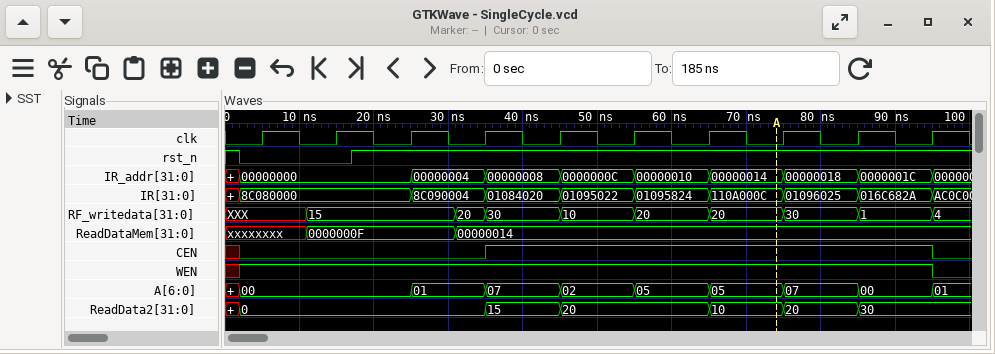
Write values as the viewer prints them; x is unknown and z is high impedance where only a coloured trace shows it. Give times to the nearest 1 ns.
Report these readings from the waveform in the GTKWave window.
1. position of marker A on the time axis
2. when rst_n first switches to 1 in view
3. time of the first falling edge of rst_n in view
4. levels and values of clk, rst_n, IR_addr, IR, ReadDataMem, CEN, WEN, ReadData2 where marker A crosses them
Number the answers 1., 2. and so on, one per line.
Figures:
1. 74 ns
2. 17 ns
3. 2 ns
4. clk=0, rst_n=1, IR_addr=00000014, IR=110A000C, ReadDataMem=00000014, CEN=1, WEN=1, ReadData2=10
